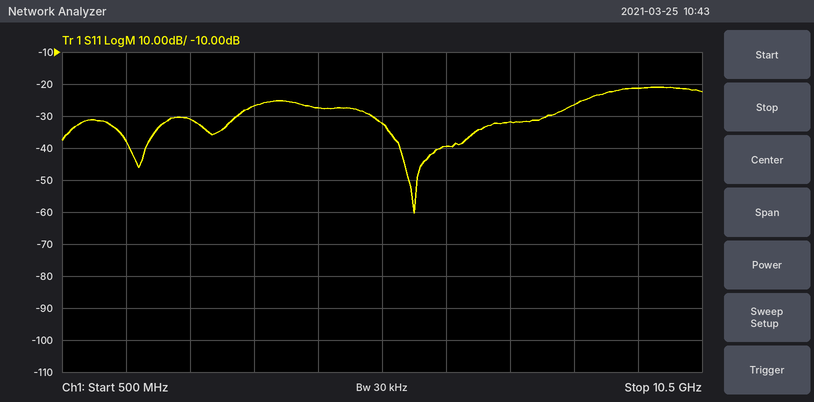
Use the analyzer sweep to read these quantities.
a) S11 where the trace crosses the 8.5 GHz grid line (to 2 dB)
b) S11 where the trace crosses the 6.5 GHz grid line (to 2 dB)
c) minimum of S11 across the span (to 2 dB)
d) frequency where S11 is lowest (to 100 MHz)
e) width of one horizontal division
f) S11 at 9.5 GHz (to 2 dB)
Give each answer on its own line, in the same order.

-26 dB
-40 dB
-60 dB
6.0 GHz
1 GHz
-22 dB
